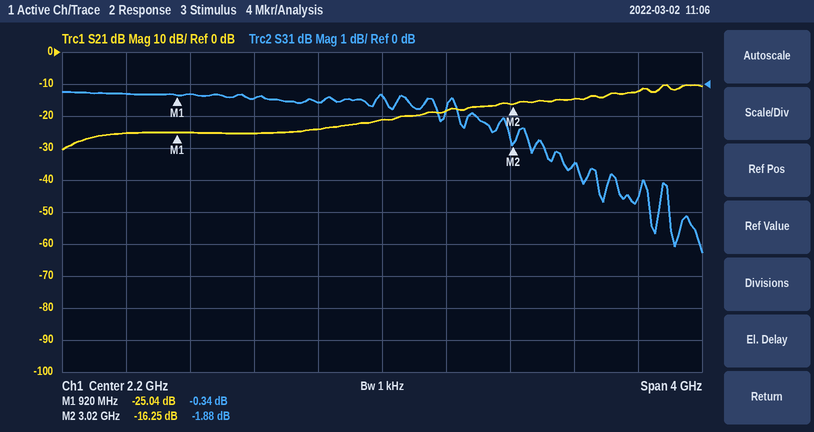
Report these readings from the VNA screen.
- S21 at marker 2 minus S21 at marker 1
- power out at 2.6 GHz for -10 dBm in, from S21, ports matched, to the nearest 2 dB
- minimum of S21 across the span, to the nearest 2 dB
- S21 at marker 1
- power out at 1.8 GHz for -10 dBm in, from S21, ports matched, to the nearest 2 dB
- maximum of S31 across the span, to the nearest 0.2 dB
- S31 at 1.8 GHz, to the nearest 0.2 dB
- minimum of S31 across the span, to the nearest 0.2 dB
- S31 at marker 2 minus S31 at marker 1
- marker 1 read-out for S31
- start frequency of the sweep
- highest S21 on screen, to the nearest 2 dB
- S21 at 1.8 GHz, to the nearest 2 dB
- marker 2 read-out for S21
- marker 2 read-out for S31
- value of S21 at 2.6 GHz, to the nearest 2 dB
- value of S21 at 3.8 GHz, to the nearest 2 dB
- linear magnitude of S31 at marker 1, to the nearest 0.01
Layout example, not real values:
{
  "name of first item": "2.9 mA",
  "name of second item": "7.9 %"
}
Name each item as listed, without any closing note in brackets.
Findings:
{
  "S21 at marker 2 minus S21 at marker 1": "8.79 dB",
  "power out at 2.6 GHz for -10 dBm in, from S21, ports matched, to the nearest 2 dB": "-28 dBm",
  "minimum of S21 across the span, to the nearest 2 dB": "-30 dB",
  "S21 at marker 1": "-25.04 dB",
  "power out at 1.8 GHz for -10 dBm in, from S21, ports matched, to the nearest 2 dB": "-34 dBm",
  "maximum of S31 across the span, to the nearest 0.2 dB": "-0.2 dB",
  "S31 at 1.8 GHz, to the nearest 0.2 dB": "-0.6 dB",
  "minimum of S31 across the span, to the nearest 0.2 dB": "-5.2 dB",
  "S31 at marker 2 minus S31 at marker 1": "-1.54 dB",
  "marker 1 read-out for S31": "-0.34 dB",
  "start frequency of the sweep": "200 MHz",
  "highest S21 on screen, to the nearest 2 dB": "-10 dB",
  "S21 at 1.8 GHz, to the nearest 2 dB": "-24 dB",
  "marker 2 read-out for S21": "-16.25 dB",
  "marker 2 read-out for S31": "-1.88 dB",
  "value of S21 at 2.6 GHz, to the nearest 2 dB": "-18 dB",
  "value of S21 at 3.8 GHz, to the nearest 2 dB": "-12 dB",
  "linear magnitude of S31 at marker 1, to the nearest 0.01": "0.96"
}
